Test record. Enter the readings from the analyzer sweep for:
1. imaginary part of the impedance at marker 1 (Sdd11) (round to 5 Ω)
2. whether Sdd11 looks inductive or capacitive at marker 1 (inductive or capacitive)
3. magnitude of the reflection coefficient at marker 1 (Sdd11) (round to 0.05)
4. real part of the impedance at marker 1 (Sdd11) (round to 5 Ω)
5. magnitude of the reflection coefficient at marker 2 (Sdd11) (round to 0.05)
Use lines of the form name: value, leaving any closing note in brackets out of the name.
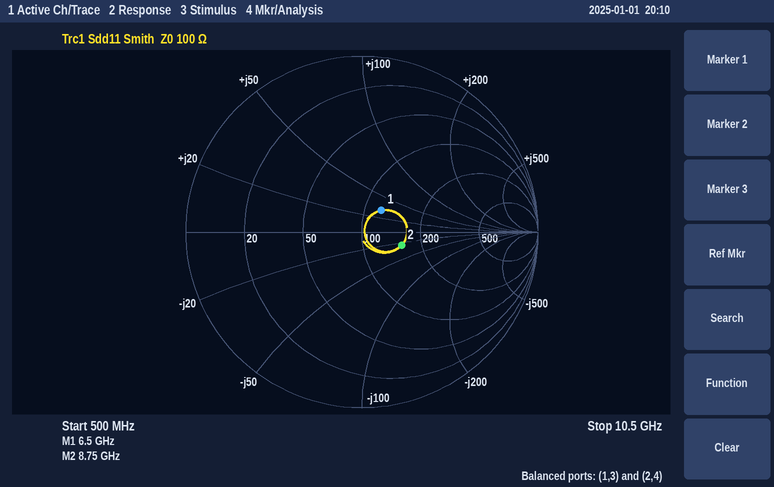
imaginary part of the impedance at marker 1 (Sdd11): +30 Ω
whether Sdd11 looks inductive or capacitive at marker 1: inductive
magnitude of the reflection coefficient at marker 1 (Sdd11): 0.15
real part of the impedance at marker 1 (Sdd11): 120 Ω
magnitude of the reflection coefficient at marker 2 (Sdd11): 0.25
